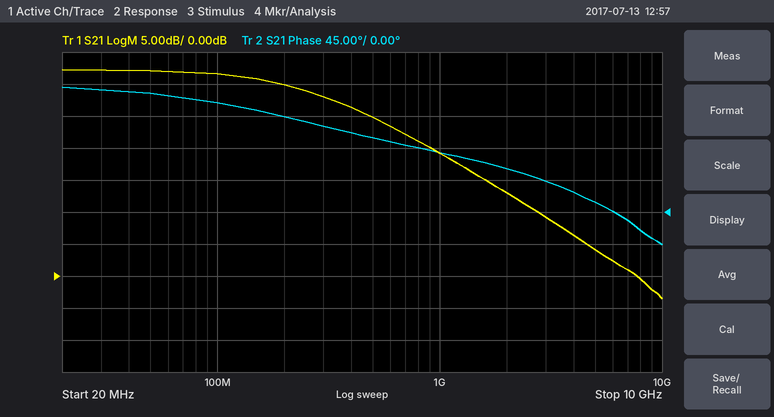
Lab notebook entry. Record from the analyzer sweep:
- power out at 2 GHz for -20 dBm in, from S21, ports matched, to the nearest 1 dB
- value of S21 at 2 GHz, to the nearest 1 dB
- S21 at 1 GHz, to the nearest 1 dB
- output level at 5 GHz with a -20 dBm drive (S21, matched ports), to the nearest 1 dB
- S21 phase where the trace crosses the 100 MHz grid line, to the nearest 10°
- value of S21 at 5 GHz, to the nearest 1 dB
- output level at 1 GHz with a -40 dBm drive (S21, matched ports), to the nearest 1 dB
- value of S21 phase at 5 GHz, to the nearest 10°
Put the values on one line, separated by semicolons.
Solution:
-7 dBm; 13 dB; 19 dB; -16 dBm; 150°; 4 dB; -21 dBm; 10°
